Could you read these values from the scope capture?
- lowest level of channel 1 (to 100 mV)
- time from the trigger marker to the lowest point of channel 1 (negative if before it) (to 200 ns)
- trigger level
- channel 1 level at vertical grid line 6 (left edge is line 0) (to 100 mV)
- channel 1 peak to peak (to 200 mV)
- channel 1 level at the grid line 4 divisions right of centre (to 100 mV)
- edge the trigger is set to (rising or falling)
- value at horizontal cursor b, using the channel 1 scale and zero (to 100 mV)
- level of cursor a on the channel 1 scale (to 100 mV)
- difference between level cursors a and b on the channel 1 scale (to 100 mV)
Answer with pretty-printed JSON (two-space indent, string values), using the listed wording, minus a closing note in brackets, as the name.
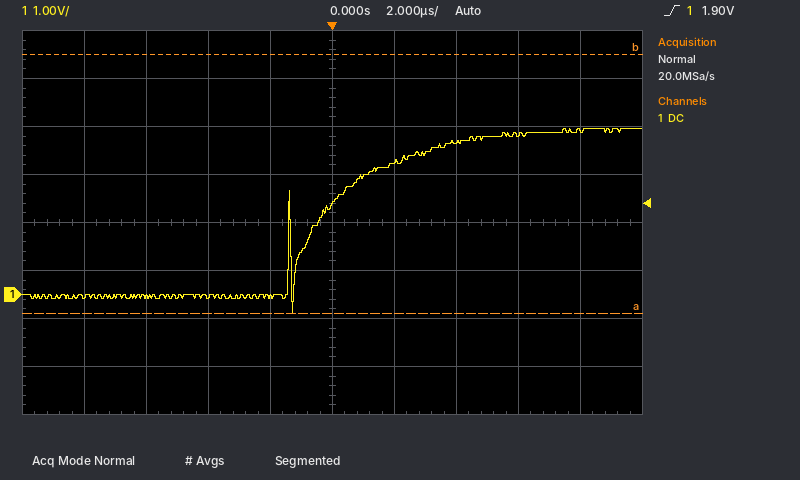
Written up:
{
  "lowest level of channel 1": "-400 mV",
  "time from the trigger marker to the lowest point of channel 1 (negative if before it)": "-1.2 µs",
  "trigger level": "1.90 V",
  "channel 1 level at vertical grid line 6 (left edge is line 0)": "2.8 V",
  "channel 1 peak to peak": "3.8 V",
  "channel 1 level at the grid line 4 divisions right of centre": "3.4 V",
  "edge the trigger is set to": "rising",
  "value at horizontal cursor b, using the channel 1 scale and zero": "5.0 V",
  "level of cursor a on the channel 1 scale": "-400 mV",
  "difference between level cursors a and b on the channel 1 scale": "5.4 V"
}
